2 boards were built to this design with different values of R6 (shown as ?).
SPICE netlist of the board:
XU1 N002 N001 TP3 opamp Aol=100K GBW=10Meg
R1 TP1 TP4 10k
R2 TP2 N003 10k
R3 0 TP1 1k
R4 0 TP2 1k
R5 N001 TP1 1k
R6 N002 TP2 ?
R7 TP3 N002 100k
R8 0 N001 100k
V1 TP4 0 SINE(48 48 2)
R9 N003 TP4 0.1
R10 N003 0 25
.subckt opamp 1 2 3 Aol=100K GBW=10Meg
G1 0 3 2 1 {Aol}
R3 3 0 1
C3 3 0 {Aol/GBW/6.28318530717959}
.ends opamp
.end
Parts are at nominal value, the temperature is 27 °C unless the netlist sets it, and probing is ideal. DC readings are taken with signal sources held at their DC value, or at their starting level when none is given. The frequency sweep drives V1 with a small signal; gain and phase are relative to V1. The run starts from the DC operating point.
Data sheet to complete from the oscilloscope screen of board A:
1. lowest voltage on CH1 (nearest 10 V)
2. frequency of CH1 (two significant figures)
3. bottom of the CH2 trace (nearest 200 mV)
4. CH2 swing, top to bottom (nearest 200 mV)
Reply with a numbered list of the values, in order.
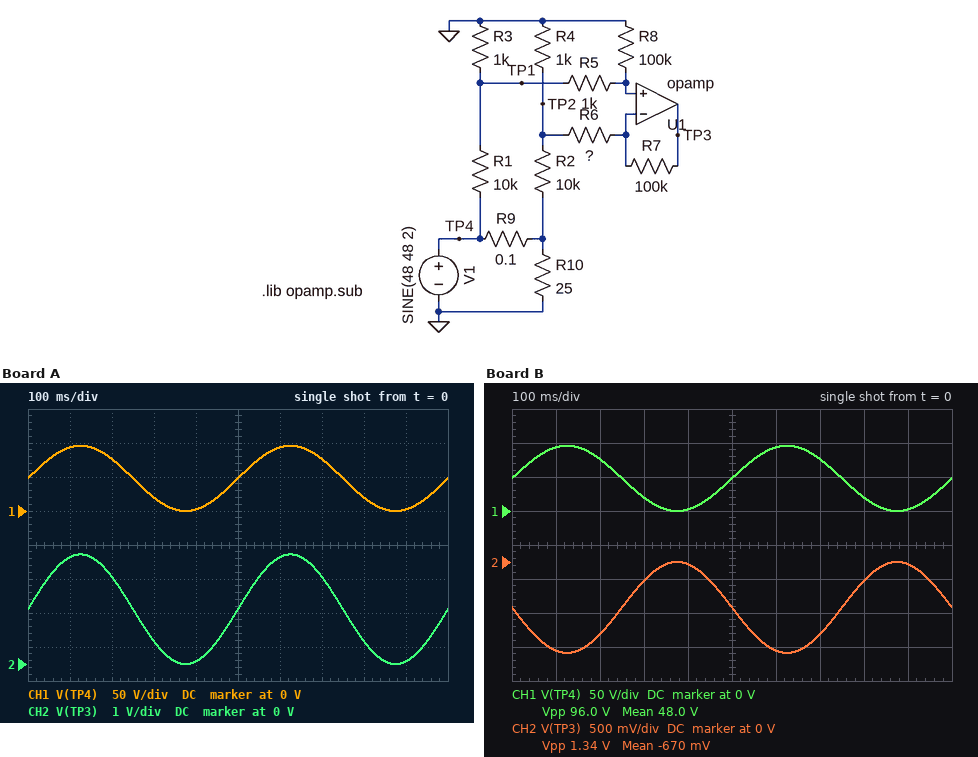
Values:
1. 0 V
2. 2.0 Hz
3. 0 V
4. 3.2 V
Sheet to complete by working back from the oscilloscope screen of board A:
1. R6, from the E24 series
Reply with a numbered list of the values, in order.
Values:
1. 1.5 kΩ
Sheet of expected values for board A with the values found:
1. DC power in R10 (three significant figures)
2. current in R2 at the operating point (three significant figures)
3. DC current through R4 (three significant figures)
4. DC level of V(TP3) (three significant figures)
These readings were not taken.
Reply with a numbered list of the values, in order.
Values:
1. 91.4 W
2. 4.35 mA
3. 4.32 mA
4. 1.61 V
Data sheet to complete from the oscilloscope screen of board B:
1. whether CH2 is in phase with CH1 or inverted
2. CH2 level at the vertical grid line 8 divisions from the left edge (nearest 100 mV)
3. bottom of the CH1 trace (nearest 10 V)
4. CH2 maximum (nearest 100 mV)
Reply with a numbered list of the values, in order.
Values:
1. inverted
2. -300 mV
3. 0 V
4. 0 V
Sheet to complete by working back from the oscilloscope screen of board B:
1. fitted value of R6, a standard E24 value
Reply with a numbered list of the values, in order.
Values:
1. 390 Ω
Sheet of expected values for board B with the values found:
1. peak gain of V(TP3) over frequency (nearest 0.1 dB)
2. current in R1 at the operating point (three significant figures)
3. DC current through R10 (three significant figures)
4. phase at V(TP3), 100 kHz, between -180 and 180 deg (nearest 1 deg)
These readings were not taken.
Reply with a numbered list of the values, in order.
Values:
1. -37.1 dB
2. 4.37 mA
3. 1.91 A
4. 142 deg
